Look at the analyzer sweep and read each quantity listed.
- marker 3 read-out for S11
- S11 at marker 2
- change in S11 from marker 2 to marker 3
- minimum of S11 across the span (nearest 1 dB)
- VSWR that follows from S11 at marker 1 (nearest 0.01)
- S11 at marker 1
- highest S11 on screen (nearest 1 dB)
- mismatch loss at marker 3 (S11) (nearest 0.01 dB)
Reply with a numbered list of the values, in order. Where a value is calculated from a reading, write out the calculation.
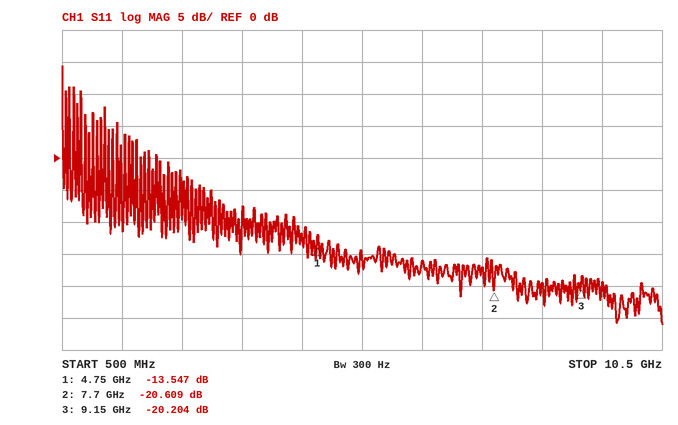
1. -20.204 dB
2. -20.609 dB
3. -20.204 − (-20.609) = 0.405 dB
4. -26 dB
5. (1 + 0.2102)/(1 − 0.2102) ≈ 1.53
6. -13.547 dB
7. 14 dB
8. −10 log10(1 − 10^(-20.204/10)) ≈ 0.04 dB
